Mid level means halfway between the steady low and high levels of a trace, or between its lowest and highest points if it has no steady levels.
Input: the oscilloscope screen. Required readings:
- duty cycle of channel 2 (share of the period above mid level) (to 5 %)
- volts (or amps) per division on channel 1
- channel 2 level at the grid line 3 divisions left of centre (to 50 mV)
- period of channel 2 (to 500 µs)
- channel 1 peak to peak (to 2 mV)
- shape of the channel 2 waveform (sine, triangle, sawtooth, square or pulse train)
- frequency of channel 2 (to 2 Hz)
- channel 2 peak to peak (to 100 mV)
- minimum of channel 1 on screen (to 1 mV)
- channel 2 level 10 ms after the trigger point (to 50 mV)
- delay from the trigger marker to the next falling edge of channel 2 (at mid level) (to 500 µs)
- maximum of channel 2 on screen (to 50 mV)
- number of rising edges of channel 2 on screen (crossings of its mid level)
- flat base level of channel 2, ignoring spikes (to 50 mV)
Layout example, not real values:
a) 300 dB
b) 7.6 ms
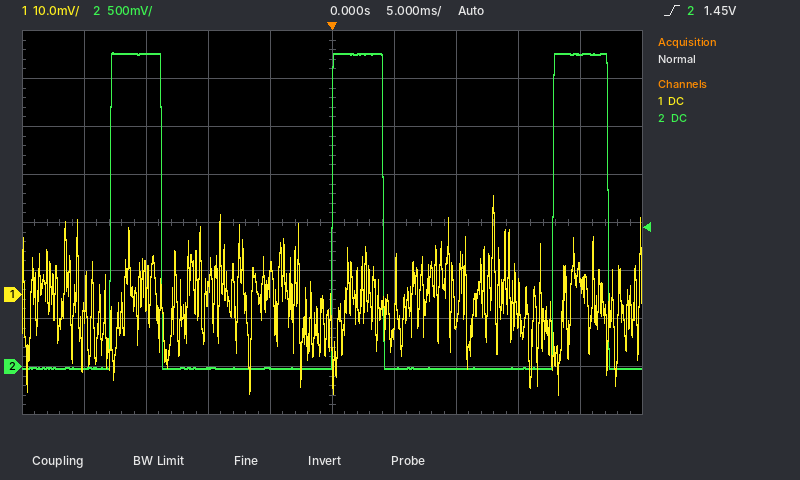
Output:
a) 25 %
b) 10 mV
c) 3.25 V
d) 18.0 ms
e) 42 mV
f) pulse train
g) 56 Hz
h) 3.30 V
i) -21 mV
j) 0 mV
k) 4.0 ms
l) 3.25 V
m) 3
n) 0 mV
